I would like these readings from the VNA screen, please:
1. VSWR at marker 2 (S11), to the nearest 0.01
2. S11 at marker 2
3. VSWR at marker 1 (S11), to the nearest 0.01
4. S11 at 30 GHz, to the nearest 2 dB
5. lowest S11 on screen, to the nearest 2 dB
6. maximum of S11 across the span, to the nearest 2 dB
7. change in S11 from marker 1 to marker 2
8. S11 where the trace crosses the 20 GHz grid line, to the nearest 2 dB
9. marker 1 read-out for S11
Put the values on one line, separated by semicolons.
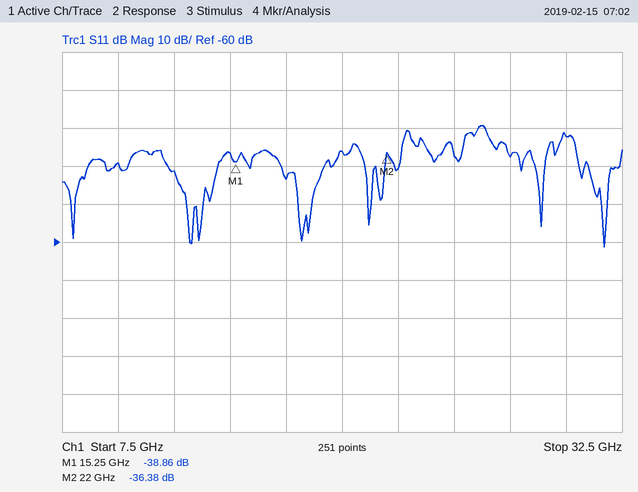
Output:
1.03; -36.38 dB; 1.02; -32 dB; -62 dB; -30 dB; 2.48 dB; -36 dB; -38.86 dB
